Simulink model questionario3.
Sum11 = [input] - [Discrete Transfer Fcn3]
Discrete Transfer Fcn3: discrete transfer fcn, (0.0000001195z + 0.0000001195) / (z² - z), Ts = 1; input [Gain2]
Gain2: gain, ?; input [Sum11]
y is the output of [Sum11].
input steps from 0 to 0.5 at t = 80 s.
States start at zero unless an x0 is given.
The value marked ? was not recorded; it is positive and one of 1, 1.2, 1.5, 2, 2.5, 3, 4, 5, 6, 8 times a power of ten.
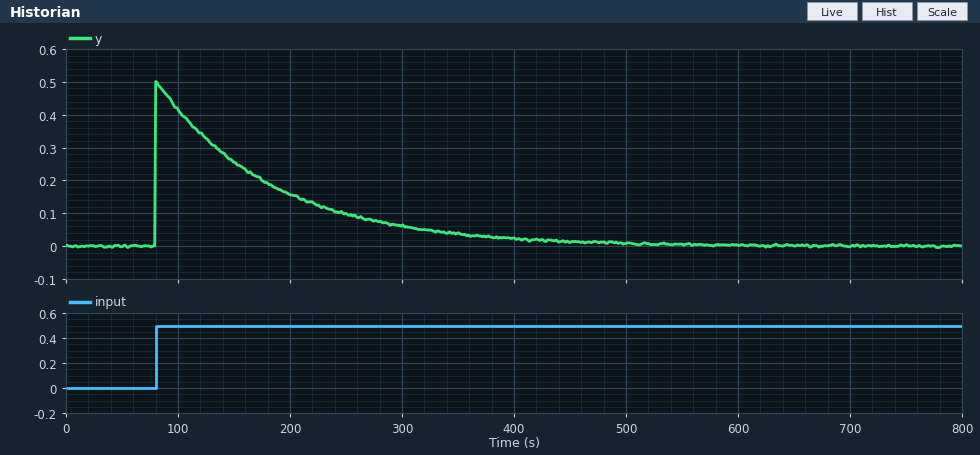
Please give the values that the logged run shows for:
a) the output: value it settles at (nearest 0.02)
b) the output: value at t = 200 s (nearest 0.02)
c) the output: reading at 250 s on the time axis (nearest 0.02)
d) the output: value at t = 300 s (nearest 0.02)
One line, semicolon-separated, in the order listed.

0.00; 0.16; 0.10; 0.06
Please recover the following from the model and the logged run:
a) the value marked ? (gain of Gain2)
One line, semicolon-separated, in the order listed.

40000
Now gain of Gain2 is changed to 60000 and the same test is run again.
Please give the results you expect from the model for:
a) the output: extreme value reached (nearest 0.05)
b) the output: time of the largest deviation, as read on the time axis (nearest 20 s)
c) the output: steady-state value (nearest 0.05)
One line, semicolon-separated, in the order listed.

0.50; 80 s; 0.00
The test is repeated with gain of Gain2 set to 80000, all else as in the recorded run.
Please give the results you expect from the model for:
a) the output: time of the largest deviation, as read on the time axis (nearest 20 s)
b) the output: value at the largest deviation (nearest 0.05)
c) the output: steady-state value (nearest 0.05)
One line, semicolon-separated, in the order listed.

80 s; 0.50; 0.00
